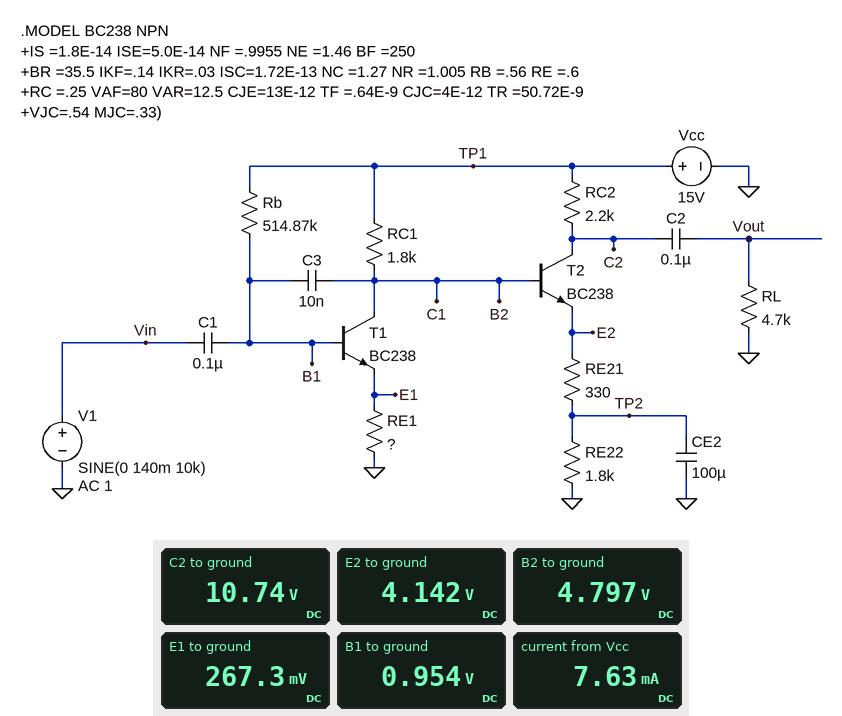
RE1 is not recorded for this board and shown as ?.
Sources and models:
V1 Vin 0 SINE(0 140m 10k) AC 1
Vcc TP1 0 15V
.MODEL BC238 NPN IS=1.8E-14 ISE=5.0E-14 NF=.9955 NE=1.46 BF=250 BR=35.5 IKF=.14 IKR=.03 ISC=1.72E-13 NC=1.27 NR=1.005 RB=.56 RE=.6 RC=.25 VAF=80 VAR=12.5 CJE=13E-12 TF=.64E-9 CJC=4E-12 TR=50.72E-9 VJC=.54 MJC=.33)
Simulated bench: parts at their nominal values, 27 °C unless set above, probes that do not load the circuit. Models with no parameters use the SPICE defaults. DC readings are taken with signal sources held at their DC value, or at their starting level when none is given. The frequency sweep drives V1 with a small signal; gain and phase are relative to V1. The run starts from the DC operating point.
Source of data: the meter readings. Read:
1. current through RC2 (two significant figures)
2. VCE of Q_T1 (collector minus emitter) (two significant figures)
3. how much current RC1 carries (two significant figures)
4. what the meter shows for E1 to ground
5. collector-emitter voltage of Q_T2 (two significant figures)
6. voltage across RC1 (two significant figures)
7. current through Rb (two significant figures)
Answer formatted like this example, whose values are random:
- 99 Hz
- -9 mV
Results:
- 1.9 mA
- 4.5 V
- 5.7 mA
- 267.3 mV
- 6.6 V
- 10 V
- 27 µA
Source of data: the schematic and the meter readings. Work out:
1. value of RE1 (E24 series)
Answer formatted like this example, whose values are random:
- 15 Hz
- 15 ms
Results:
- 47 Ω
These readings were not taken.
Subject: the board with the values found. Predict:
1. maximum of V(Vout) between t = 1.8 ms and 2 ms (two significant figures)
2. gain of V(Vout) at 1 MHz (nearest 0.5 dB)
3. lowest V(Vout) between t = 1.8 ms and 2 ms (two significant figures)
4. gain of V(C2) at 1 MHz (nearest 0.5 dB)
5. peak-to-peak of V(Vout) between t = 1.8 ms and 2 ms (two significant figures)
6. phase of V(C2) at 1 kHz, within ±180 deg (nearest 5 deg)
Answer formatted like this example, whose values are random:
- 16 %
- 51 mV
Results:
- 3.2 V
- 13.0 dB
- -4.2 V
- 13.0 dB
- 7.4 V
- -5 deg
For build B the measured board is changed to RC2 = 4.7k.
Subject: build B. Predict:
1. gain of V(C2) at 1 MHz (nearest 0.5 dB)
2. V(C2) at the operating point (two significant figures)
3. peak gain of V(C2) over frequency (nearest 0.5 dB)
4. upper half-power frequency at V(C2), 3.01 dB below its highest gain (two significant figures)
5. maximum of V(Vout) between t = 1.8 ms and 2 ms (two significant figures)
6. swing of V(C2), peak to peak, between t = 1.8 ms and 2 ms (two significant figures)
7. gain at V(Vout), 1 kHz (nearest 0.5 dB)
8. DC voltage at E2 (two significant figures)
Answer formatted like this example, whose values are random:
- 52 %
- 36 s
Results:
- 17.0 dB
- 5.9 V
- 38.5 dB
- 420 Hz
- 3.7 V
- 6.9 V
- 34.0 dB
- 4.1 V
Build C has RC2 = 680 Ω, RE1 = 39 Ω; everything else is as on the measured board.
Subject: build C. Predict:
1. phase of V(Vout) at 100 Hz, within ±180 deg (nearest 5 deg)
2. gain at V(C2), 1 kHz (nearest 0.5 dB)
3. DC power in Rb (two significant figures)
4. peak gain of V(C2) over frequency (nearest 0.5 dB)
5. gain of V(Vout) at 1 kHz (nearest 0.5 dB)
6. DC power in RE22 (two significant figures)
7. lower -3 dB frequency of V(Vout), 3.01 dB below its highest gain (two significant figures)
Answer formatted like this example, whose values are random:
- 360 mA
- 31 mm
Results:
- 95 deg
- 22.5 dB
- 390 µW
- 23.0 dB
- 22.0 dB
- 6.7 mW
- 300 Hz
